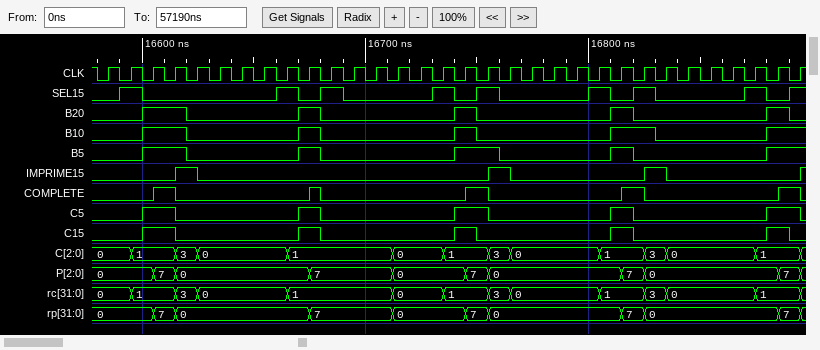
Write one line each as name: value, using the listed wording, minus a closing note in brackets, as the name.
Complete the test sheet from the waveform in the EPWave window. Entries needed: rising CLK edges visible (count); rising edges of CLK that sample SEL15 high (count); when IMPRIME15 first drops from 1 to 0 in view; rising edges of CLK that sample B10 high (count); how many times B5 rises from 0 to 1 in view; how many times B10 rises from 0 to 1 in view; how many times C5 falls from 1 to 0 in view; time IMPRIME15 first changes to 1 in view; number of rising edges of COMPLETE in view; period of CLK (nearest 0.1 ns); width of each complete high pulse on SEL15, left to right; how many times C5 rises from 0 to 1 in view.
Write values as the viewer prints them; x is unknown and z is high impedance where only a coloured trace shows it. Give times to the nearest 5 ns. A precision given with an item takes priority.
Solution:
rising CLK edges visible: 32
rising edges of CLK that sample SEL15 high: 9
when IMPRIME15 first drops from 1 to 0 in view: 16625 ns
rising edges of CLK that sample B10 high: 8
how many times B5 rises from 0 to 1 in view: 5
how many times B10 rises from 0 to 1 in view: 5
how many times C5 falls from 1 to 0 in view: 5
time IMPRIME15 first changes to 1 in view: 16615 ns
number of rising edges of COMPLETE in view: 5
period of CLK: 10 ns
width of each complete high pulse on SEL15, left to right: 10 ns, 10 ns, 10 ns, 10 ns, 10 ns, 10 ns, 10 ns, 10 ns
how many times C5 rises from 0 to 1 in view: 5
